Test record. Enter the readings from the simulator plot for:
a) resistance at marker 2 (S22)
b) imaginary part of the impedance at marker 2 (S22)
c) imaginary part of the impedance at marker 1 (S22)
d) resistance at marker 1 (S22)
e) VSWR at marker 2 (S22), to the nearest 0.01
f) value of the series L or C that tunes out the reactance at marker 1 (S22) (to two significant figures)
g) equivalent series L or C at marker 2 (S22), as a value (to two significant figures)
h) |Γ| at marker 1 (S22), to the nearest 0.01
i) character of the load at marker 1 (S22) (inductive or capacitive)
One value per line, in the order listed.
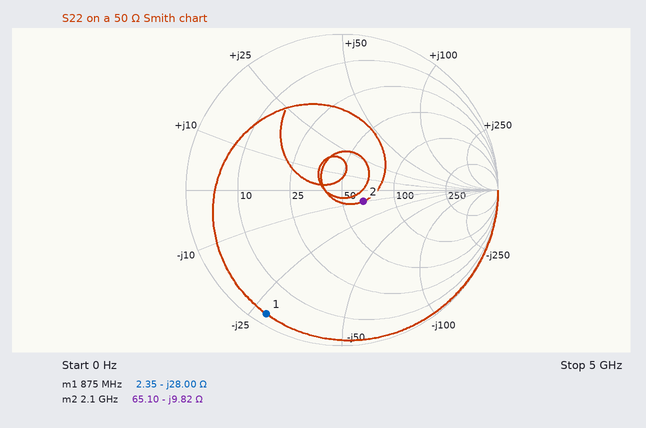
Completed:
65.10 Ω
-9.82 Ω
-28.00 Ω
2.35 Ω
1.37
5.1 nH
7.7 pF
0.93
capacitive
